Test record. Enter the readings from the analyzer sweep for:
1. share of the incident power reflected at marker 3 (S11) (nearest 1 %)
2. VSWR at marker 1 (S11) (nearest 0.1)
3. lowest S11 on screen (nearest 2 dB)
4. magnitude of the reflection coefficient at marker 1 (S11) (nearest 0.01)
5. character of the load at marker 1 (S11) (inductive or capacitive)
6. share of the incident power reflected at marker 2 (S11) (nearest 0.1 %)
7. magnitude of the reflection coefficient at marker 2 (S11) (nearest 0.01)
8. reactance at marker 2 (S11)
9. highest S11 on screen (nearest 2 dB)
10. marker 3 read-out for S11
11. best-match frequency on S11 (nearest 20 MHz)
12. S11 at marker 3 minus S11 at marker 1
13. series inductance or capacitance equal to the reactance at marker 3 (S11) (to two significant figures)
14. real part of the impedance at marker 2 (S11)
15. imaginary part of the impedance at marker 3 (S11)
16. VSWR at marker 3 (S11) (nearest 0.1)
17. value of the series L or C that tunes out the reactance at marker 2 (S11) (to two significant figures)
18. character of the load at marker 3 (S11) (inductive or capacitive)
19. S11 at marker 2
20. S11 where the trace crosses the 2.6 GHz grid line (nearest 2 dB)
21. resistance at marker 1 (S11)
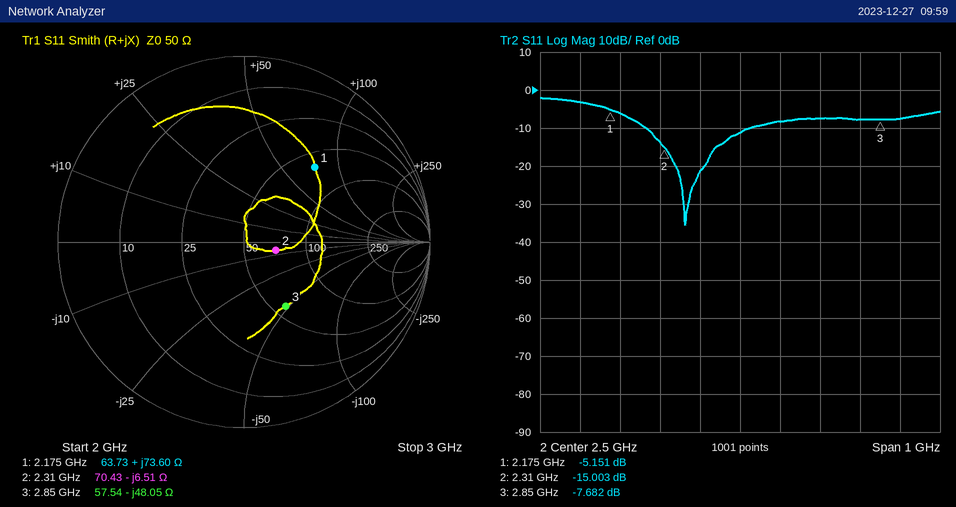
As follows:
17 %
3.5
-36 dB
0.55
inductive
3.2 %
0.18
-6.51 Ω
-2 dB
-7.682 dB
2.36 GHz
-2.531 dB
1.2 pF
70.43 Ω
-48.05 Ω
2.4
450 pH
capacitive
-15.003 dB
-8 dB
63.73 Ω
